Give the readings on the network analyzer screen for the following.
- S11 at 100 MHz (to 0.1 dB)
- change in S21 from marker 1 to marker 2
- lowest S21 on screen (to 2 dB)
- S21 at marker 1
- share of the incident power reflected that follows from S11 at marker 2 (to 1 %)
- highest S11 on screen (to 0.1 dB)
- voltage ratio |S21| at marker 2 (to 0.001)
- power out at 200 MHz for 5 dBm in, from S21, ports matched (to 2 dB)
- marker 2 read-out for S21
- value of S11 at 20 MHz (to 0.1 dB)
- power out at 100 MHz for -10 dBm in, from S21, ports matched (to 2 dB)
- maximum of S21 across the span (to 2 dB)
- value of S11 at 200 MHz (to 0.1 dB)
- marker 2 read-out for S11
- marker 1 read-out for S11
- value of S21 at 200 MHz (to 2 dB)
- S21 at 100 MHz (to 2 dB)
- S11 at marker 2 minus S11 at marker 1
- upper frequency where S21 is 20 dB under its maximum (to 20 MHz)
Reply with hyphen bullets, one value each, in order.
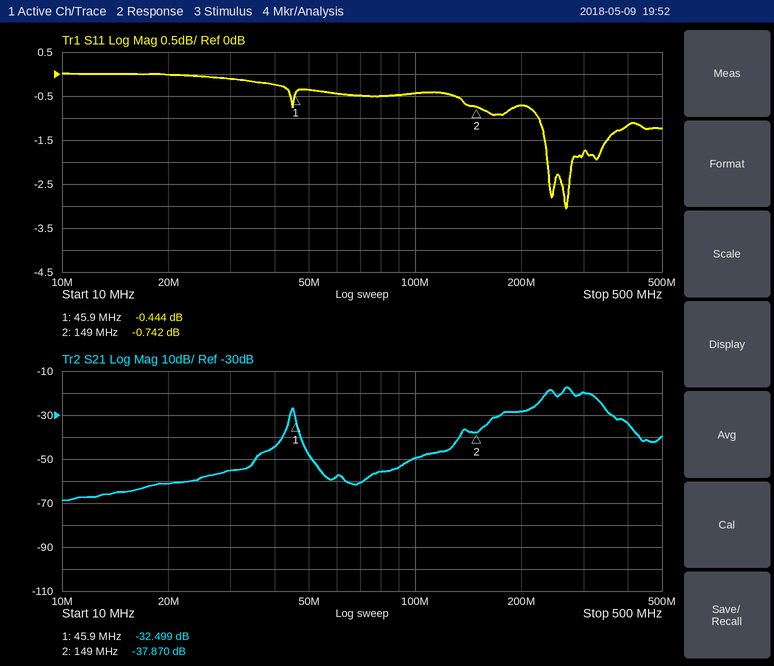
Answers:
- -0.4 dB
- -5.371 dB
- -68 dB
- -32.499 dB
- 84 %
- 0.0 dB
- 0.013
- -24 dBm
- -37.870 dB
- 0.0 dB
- -60 dBm
- -18 dB
- -0.7 dB
- -0.742 dB
- -0.444 dB
- -28 dB
- -50 dB
- -0.298 dB
- 420 MHz
